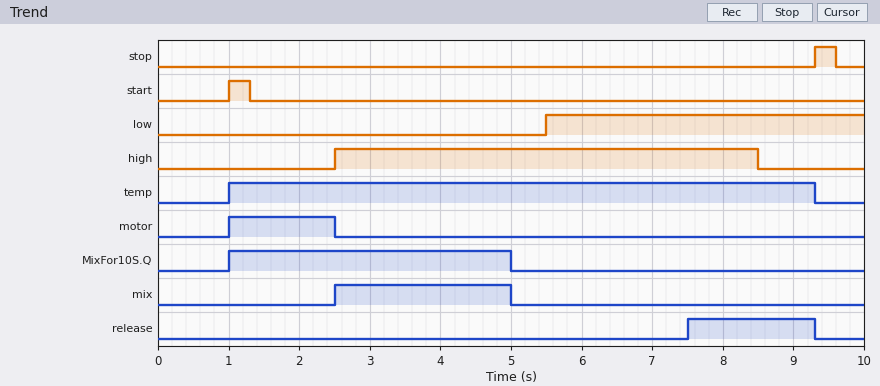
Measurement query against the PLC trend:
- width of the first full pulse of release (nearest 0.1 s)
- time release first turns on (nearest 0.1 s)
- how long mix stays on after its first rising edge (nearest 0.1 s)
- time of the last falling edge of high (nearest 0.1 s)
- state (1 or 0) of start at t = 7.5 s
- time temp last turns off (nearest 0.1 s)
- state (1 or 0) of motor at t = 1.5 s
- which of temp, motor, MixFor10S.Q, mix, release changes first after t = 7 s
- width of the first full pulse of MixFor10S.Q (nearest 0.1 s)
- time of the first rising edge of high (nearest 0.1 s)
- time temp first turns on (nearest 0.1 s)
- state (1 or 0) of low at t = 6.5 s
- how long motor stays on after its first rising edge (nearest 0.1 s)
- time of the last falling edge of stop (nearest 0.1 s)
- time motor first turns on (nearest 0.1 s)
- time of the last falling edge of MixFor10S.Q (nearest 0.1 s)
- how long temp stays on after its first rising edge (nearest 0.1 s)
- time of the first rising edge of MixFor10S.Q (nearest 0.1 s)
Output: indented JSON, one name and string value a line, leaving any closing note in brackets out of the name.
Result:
{
  "width of the first full pulse of release": "1.8 s",
  "time release first turns on": "7.5 s",
  "how long mix stays on after its first rising edge": "2.5 s",
  "time of the last falling edge of high": "8.5 s",
  "state (1 or 0) of start at t = 7.5 s": "0",
  "time temp last turns off": "9.3 s",
  "state (1 or 0) of motor at t = 1.5 s": "1",
  "which of temp, motor, MixFor10S.Q, mix, release changes first after t = 7 s": "release",
  "width of the first full pulse of MixFor10S.Q": "4.0 s",
  "time of the first rising edge of high": "2.5 s",
  "time temp first turns on": "1.0 s",
  "state (1 or 0) of low at t = 6.5 s": "1",
  "how long motor stays on after its first rising edge": "1.5 s",
  "time of the last falling edge of stop": "9.6 s",
  "time motor first turns on": "1.0 s",
  "time of the last falling edge of MixFor10S.Q": "5.0 s",
  "how long temp stays on after its first rising edge": "8.3 s",
  "time of the first rising edge of MixFor10S.Q": "1.0 s"
}
